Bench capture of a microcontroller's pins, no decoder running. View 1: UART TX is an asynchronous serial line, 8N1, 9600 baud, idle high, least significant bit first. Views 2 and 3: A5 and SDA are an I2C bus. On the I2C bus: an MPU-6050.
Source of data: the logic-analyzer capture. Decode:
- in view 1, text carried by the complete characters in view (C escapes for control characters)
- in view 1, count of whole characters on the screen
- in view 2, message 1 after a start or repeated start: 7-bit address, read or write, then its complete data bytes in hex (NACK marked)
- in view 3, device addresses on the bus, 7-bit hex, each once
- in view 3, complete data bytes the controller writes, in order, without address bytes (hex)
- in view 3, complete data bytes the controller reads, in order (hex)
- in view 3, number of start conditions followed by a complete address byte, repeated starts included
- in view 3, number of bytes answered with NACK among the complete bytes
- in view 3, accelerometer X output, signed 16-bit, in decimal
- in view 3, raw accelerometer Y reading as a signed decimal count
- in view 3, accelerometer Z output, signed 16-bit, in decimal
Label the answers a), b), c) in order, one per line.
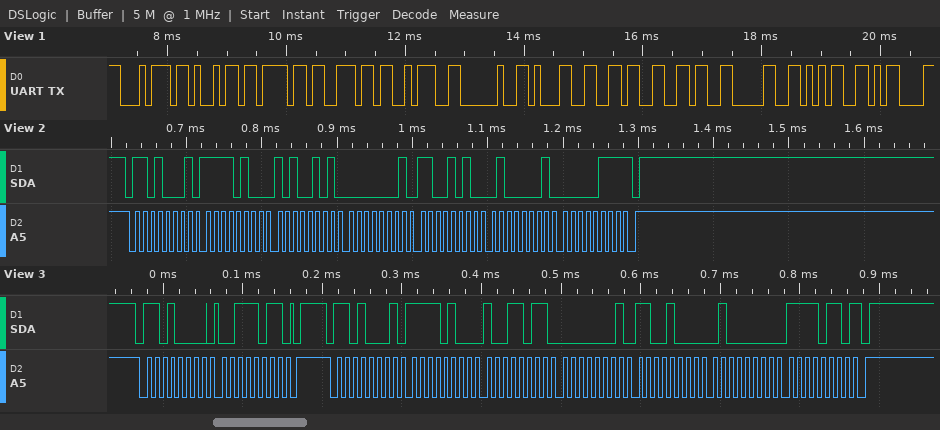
a) "tion: 16605\r"
b) 12
c) 0x68 read: F4 A5 01 CA 41 07 NACK
d) 0x68
e) 3B
f) F4 9B 01 C8 40 F6
g) 2
h) 1
i) -2917
j) 456
k) 16630
